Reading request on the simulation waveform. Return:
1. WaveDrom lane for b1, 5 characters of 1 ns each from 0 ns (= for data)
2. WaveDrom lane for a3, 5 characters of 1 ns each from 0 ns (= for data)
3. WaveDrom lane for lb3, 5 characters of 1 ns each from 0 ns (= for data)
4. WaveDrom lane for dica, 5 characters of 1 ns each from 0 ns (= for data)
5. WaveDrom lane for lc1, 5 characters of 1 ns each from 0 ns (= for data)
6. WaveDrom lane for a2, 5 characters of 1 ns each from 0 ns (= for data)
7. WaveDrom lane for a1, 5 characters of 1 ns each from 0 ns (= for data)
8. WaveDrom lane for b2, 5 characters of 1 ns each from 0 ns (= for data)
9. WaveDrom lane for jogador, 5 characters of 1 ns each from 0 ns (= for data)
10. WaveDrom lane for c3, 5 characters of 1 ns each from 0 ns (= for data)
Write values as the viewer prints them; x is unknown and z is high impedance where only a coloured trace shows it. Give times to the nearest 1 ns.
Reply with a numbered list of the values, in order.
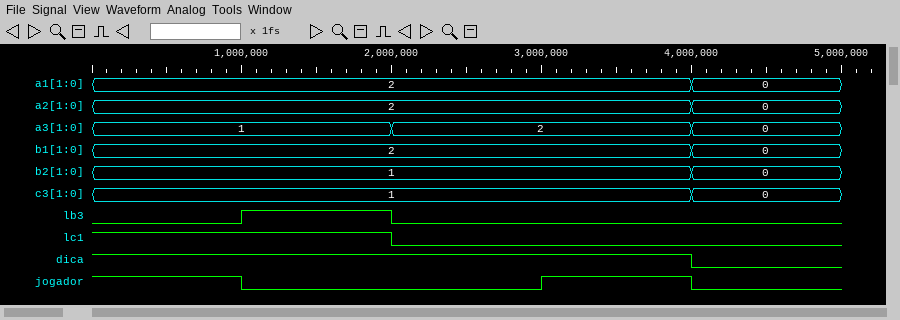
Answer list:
1. {name: 'b1', wave: '=...=', data: '2 0'}
2. {name: 'a3', wave: '=.=.=', data: '1 2 0'}
3. {name: 'lb3', wave: '010..'}
4. {name: 'dica', wave: '1...0'}
5. {name: 'lc1', wave: '1.0..'}
6. {name: 'a2', wave: '=...=', data: '2 0'}
7. {name: 'a1', wave: '=...=', data: '2 0'}
8. {name: 'b2', wave: '=...=', data: '1 0'}
9. {name: 'jogador', wave: '10.10'}
10. {name: 'c3', wave: '=...=', data: '1 0'}
